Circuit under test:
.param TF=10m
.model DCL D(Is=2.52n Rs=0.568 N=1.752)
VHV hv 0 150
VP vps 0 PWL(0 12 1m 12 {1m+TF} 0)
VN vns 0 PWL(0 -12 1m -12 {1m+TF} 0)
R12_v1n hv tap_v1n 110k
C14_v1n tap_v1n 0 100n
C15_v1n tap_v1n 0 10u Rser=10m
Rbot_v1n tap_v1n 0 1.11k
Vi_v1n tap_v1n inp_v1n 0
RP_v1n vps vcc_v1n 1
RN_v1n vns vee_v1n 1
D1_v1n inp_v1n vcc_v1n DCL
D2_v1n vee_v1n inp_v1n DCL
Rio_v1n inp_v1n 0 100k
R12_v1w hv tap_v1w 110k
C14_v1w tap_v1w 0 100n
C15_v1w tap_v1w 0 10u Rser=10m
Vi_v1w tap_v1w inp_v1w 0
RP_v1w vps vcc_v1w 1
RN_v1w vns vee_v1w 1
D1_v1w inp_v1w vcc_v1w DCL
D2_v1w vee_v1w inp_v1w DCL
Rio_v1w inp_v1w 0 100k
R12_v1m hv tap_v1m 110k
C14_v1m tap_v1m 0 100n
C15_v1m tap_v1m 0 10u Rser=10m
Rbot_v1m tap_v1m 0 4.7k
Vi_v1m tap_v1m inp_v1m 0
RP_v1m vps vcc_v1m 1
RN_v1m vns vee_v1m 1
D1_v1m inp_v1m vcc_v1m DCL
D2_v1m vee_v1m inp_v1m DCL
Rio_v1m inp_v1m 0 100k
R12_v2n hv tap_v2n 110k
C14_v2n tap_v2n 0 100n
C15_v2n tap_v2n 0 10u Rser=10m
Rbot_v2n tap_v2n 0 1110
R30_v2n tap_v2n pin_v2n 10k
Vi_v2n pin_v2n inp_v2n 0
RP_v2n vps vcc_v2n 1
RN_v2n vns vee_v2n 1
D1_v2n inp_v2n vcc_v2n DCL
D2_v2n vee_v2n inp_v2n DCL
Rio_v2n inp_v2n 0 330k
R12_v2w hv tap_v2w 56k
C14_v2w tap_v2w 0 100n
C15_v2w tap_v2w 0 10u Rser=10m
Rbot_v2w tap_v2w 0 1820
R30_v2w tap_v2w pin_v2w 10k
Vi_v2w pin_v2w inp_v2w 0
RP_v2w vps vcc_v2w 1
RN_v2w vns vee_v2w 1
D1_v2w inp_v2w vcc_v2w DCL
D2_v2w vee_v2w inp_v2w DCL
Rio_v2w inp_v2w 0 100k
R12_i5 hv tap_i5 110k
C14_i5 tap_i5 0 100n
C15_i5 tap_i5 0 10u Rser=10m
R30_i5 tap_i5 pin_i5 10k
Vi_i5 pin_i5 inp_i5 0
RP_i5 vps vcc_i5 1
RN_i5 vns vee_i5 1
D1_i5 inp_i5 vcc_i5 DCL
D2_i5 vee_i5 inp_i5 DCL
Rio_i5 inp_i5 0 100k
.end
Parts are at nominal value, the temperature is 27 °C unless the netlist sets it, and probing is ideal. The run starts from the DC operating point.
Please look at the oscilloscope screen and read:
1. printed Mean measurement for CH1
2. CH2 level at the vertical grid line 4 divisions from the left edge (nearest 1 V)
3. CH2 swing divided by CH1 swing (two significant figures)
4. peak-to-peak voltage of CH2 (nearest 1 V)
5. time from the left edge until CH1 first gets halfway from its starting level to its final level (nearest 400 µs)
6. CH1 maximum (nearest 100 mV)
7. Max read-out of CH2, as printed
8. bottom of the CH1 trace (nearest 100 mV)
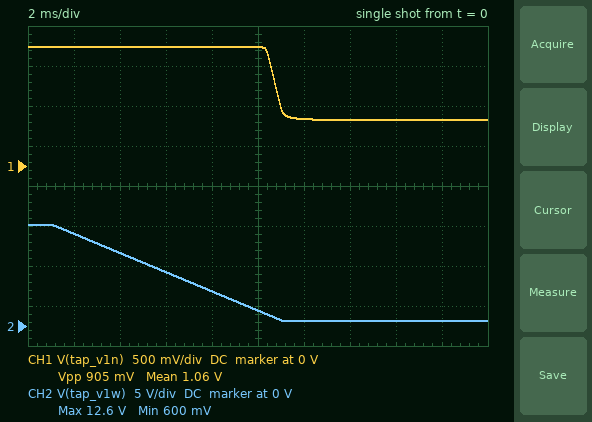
1.06 V
4 V
13
12 V
10.8 ms
1.5 V
12.6 V
600 mV
